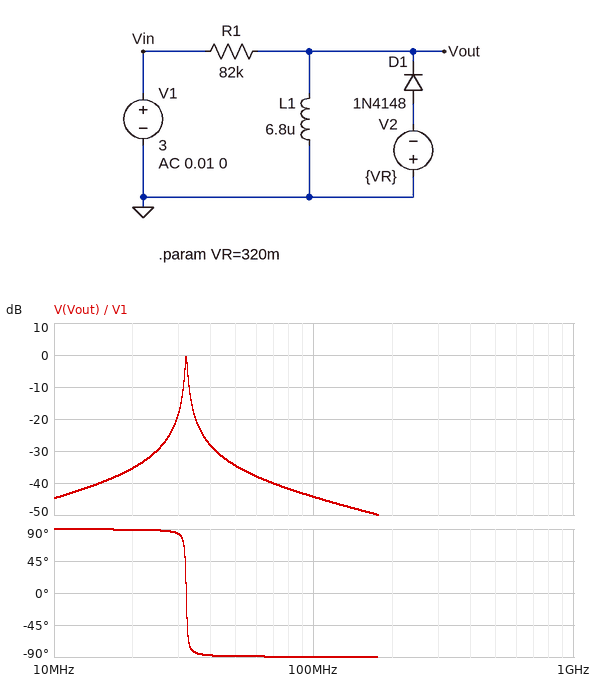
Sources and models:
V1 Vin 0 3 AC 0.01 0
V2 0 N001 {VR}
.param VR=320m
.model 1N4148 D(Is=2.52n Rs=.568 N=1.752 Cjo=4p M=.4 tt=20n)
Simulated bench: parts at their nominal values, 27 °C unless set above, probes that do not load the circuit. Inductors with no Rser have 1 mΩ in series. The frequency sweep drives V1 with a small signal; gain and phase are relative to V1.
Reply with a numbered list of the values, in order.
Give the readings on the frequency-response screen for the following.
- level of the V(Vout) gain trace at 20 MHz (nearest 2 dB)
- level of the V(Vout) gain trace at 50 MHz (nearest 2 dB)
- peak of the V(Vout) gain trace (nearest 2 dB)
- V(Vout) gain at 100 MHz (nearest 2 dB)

1. -36 dB
2. -34 dB
3. 0 dB
4. -44 dB
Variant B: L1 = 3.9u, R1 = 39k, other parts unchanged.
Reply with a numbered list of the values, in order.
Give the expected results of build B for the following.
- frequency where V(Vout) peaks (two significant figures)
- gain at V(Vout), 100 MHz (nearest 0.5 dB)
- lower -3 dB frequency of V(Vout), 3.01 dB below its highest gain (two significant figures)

1. 43 MHz
2. -37.0 dB
3. 42 MHz
